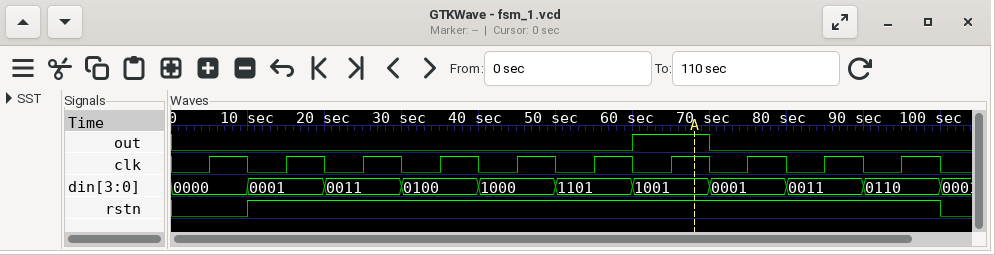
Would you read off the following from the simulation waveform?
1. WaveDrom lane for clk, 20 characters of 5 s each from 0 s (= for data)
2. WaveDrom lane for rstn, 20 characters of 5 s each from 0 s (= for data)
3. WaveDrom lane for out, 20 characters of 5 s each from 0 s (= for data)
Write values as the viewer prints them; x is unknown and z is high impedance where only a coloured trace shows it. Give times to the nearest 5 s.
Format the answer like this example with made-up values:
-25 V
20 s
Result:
{name: 'clk', wave: '01010101010101010101'}
{name: 'rstn', wave: '0.1.................'}
{name: 'out', wave: '0...........1.0.....'}
